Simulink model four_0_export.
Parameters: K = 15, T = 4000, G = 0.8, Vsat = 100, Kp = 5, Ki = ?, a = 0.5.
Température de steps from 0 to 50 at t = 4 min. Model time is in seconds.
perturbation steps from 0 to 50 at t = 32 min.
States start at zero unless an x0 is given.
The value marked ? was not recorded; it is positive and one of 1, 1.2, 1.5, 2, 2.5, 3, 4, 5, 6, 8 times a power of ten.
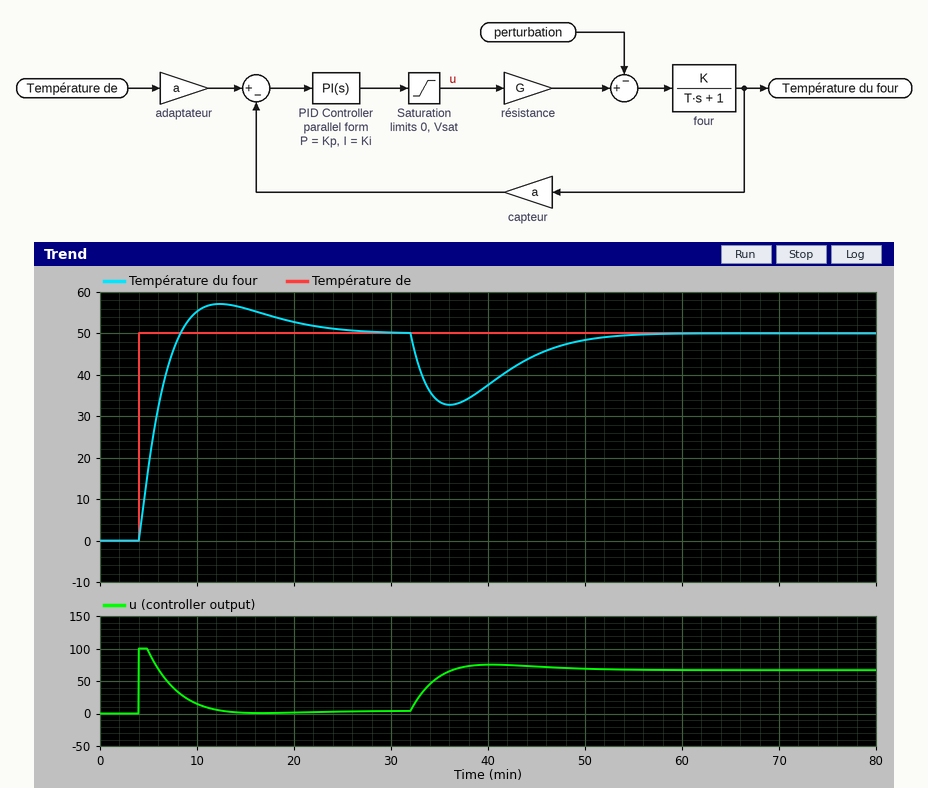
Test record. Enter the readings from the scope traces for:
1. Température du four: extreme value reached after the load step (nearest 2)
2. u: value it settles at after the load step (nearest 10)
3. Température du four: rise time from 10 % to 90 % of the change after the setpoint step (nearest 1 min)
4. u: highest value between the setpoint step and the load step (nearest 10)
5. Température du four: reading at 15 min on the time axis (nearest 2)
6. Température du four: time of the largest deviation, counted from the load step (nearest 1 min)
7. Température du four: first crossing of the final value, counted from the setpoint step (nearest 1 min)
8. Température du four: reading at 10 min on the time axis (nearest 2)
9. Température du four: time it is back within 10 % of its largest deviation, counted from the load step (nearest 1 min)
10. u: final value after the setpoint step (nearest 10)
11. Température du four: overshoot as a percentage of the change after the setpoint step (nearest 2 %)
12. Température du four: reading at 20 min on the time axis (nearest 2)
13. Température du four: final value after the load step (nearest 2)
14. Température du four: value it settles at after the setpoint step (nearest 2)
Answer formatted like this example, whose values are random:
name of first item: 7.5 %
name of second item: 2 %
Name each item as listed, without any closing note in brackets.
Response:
Température du four: extreme value reached after the load step: 32
u: value it settles at after the load step: 70
Température du four: rise time from 10 % to 90 % of the change after the setpoint step: 3 min
u: highest value between the setpoint step and the load step: 100
Température du four: reading at 15 min on the time axis: 56
Température du four: time of the largest deviation, counted from the load step: 4 min
Température du four: first crossing of the final value, counted from the setpoint step: 4 min
Température du four: reading at 10 min on the time axis: 56
Température du four: time it is back within 10 % of its largest deviation, counted from the load step: 18 min
u: final value after the setpoint step: 0
Température du four: overshoot as a percentage of the change after the setpoint step: 14 %
Température du four: reading at 20 min on the time axis: 52
Température du four: final value after the load step: 50
Température du four: value it settles at after the setpoint step: 50
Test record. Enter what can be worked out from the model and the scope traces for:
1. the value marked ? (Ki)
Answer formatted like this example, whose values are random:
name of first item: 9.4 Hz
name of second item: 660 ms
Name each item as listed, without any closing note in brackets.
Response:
the value marked ?: 0.012
